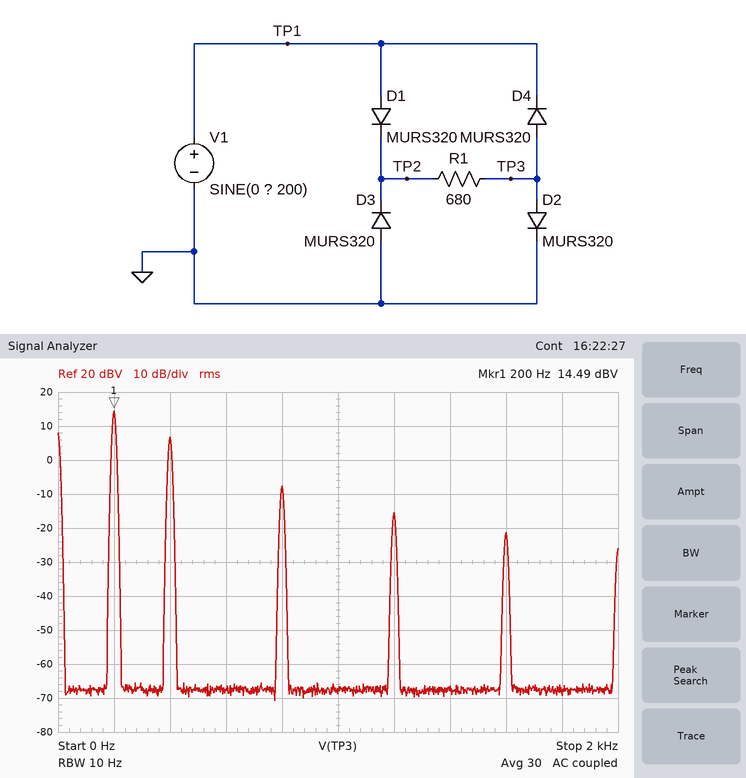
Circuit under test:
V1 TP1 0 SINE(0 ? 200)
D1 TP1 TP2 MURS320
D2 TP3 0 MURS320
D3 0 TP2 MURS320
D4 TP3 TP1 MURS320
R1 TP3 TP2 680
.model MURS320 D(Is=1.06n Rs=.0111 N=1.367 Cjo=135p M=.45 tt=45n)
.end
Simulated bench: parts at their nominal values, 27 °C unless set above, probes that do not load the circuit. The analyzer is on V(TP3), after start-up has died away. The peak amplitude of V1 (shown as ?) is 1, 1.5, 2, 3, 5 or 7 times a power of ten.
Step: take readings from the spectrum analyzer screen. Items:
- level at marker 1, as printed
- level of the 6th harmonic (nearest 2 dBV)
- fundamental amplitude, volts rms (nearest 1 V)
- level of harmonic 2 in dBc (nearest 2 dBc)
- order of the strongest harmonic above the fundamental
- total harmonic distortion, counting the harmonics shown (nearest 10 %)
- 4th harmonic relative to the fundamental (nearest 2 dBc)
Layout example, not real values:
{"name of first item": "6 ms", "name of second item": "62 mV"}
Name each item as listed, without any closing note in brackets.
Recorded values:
{"level at marker 1, as printed": "14.49 dBV", "level of the 6th harmonic": "-16 dBV", "fundamental amplitude, volts rms": "5 V", "level of harmonic 2 in dBc": "-8 dBc", "order of the strongest harmonic above the fundamental": "2", "total harmonic distortion, counting the harmonics shown": "40 %", "4th harmonic relative to the fundamental": "-22 dBc"}
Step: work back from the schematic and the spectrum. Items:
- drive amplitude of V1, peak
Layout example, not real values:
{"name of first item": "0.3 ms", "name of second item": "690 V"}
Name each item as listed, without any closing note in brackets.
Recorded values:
{"drive amplitude of V1, peak": "15 V"}
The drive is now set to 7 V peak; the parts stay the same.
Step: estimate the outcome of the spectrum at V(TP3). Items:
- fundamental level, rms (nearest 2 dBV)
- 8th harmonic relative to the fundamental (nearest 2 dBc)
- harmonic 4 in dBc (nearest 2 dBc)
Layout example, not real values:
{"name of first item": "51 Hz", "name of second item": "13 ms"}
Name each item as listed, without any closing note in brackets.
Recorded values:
{"fundamental level, rms": "8 dBV", "8th harmonic relative to the fundamental": "-42 dBc", "harmonic 4 in dBc": "-24 dBc"}
